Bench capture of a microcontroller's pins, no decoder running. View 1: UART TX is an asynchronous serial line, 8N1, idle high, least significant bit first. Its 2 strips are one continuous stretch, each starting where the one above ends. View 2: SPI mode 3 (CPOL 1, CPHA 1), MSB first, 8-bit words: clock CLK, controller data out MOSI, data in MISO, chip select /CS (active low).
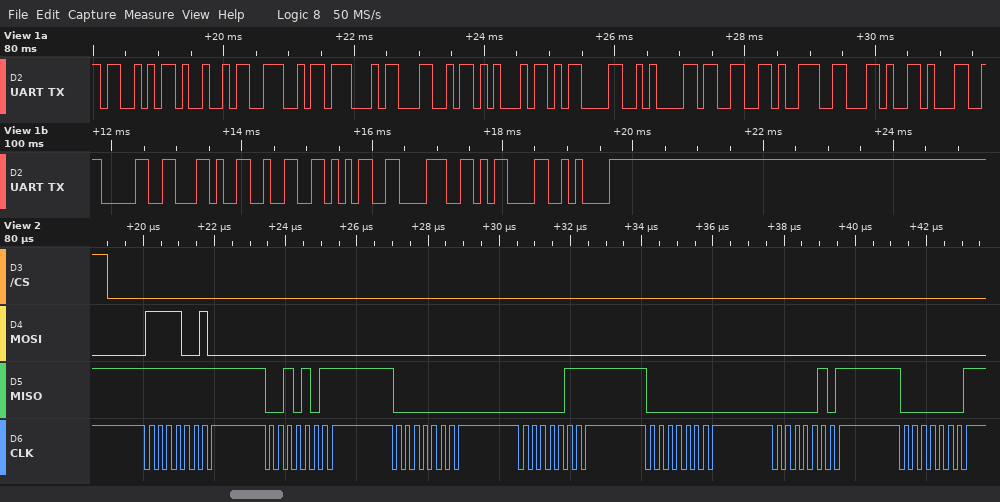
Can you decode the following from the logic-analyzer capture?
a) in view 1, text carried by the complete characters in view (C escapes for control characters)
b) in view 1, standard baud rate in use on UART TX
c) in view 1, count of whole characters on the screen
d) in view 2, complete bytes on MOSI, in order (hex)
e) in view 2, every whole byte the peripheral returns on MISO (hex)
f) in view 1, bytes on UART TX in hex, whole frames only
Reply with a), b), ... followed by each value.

a) "SINGLE\r\n39,10,258\r\n"
b) 9600 baud
c) 19
d) F2 00 00 00 00 00 00
e) FF 2B 00 07 00 05 01
f) 53 49 4E 47 4C 45 0D 0A 33 39 2C 31 30 2C 32 35 38 0D 0A
